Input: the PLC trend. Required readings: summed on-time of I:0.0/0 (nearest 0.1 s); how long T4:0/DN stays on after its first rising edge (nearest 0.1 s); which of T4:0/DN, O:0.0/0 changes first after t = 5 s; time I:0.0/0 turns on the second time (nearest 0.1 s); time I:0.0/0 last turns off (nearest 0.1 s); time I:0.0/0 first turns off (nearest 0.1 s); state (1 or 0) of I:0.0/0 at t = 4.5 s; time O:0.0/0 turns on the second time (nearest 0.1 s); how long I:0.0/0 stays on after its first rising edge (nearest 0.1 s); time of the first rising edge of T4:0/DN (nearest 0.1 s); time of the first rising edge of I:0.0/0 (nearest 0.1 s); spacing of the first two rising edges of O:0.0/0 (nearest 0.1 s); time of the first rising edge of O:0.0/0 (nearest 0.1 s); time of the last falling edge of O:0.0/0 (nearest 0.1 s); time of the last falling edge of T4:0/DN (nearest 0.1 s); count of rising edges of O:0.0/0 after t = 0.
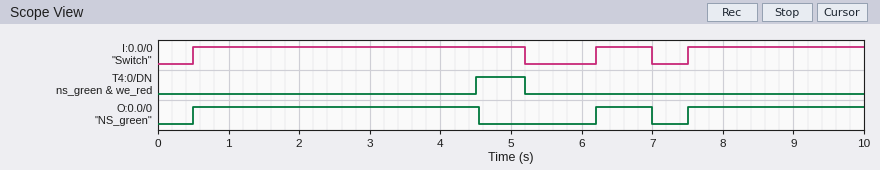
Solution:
8.0 s
0.7 s
T4:0/DN
6.2 s
7.0 s
5.2 s
1
6.2 s
4.7 s
4.5 s
0.5 s
5.7 s
0.5 s
7.0 s
5.2 s
3
